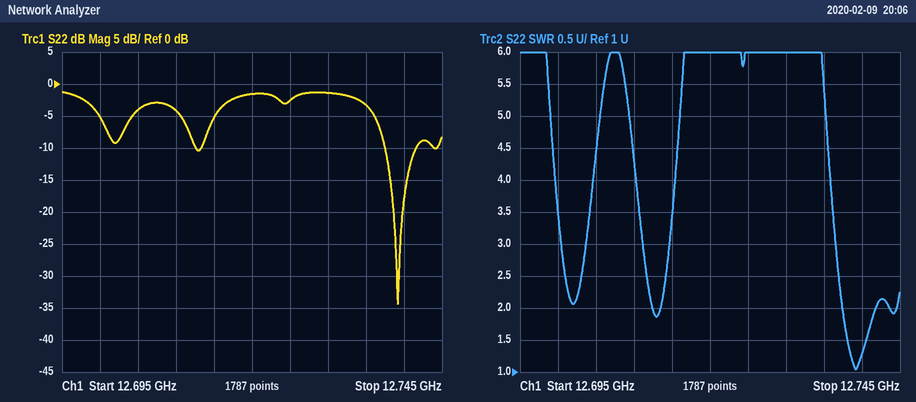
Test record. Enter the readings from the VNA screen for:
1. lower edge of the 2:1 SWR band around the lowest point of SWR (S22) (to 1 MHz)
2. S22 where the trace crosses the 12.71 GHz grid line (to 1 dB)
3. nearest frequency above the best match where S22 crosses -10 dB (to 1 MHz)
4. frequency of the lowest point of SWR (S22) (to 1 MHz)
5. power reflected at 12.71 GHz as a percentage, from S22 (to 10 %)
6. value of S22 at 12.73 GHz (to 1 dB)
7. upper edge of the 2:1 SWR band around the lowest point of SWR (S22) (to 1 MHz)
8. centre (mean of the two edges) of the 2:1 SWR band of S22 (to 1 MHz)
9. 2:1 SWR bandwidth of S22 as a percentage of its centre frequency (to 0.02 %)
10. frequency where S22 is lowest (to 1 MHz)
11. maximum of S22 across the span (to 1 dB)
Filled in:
12.737 GHz
-4 dB
12.742 GHz
12.739 GHz
40 %
-1 dB
12.742 GHz
12.740 GHz
0.04 %
12.739 GHz
-1 dB
